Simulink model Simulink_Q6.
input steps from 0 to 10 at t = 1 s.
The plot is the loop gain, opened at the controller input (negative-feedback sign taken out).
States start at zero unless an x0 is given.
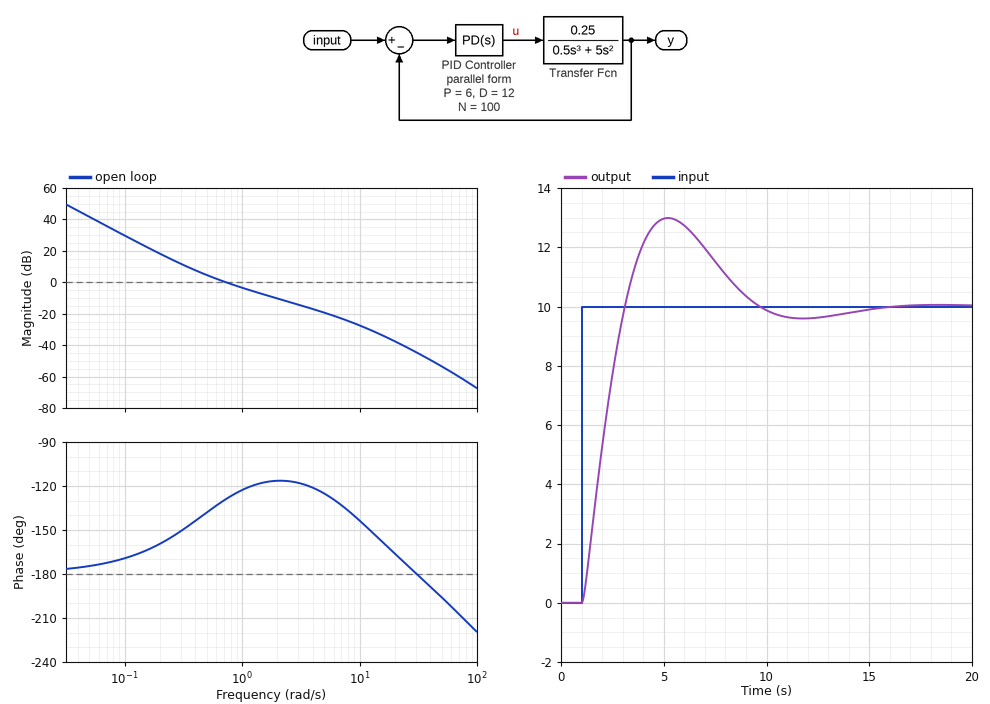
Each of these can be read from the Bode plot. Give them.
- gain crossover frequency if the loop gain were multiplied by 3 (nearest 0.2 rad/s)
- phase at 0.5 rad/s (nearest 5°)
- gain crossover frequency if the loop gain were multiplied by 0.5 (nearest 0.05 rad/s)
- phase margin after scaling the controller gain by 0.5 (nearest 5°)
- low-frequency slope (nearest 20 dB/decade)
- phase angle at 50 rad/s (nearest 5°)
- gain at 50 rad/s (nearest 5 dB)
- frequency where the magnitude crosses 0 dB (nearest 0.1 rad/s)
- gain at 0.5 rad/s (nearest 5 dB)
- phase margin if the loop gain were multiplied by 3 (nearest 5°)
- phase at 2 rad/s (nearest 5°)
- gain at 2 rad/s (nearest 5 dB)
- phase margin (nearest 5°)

1.8 rad/s
-140°
0.45 rad/s
40°
-40 dB/decade
-195°
-55 dB
0.7 rad/s
5 dB
65°
-115°
-10 dB
50°
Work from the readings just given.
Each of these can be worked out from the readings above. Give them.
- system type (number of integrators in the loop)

2
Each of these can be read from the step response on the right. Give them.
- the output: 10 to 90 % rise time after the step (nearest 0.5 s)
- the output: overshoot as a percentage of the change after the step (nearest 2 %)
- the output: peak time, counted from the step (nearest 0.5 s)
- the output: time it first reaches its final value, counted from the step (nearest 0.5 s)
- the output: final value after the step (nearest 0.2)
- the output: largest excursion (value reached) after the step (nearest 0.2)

1.5 s
30 %
4.0 s
2.0 s
10.0
13.0
